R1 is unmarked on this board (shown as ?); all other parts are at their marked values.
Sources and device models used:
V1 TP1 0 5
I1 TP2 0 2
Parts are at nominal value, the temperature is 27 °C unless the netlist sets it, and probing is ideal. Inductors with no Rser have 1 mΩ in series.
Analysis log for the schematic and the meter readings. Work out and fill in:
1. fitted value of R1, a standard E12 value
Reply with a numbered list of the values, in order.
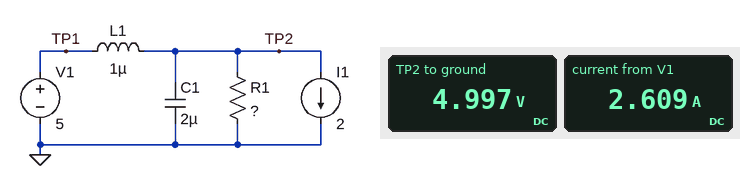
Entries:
1. 8.2 Ω
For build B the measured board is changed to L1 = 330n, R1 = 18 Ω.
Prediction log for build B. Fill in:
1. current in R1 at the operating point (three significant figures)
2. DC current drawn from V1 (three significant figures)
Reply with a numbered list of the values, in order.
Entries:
1. 278 mA
2. 2.28 A
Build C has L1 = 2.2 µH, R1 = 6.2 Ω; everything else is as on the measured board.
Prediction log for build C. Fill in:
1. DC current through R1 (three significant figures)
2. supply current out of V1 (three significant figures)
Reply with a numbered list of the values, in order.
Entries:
1. 806 mA
2. 2.81 A
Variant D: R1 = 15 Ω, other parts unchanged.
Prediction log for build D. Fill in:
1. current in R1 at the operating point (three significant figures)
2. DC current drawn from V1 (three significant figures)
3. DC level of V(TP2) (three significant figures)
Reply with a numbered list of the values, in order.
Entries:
1. 333 mA
2. 2.33 A
3. 5.00 V
